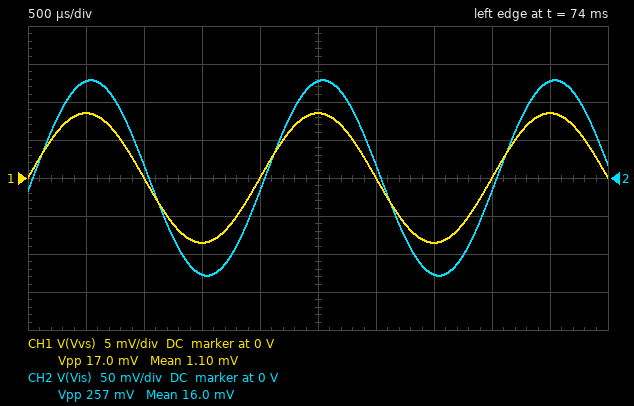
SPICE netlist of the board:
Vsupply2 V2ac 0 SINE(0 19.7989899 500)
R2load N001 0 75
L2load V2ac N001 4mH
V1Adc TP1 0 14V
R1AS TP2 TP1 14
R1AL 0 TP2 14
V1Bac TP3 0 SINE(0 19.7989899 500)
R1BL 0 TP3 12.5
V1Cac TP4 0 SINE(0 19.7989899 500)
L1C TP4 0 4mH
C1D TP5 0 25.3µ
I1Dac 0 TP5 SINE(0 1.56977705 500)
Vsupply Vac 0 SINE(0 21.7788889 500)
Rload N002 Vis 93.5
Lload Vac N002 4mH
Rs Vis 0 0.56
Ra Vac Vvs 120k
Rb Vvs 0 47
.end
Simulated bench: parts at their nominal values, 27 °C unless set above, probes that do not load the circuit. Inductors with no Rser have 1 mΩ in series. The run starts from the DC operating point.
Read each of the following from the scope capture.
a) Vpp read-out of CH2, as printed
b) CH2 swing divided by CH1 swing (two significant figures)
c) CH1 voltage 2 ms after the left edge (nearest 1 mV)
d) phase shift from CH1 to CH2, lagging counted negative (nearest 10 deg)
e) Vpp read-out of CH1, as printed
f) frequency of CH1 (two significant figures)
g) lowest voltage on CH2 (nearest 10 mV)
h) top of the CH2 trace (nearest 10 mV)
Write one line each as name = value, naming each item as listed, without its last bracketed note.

Vpp read-out of CH2, as printed = 257 mV
CH2 swing divided by CH1 swing = 15
CH1 voltage 2 ms after the left edge = 0 V
phase shift from CH1 to CH2, lagging counted negative = -10 deg
Vpp read-out of CH1, as printed = 17.0 mV
frequency of CH1 = 500 Hz
lowest voltage on CH2 = -130 mV
top of the CH2 trace = 130 mV
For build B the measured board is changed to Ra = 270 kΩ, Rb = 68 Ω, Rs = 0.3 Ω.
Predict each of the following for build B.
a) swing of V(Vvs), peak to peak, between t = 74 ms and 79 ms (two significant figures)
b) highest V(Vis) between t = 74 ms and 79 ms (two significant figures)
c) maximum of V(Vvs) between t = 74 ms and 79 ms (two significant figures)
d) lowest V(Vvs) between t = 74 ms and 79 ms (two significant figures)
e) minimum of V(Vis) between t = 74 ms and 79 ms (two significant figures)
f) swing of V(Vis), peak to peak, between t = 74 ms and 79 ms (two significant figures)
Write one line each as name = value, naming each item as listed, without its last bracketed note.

swing of V(Vvs), peak to peak, between t = 74 ms and 79 ms = 11 mV
highest V(Vis) between t = 74 ms and 79 ms = 69 mV
maximum of V(Vvs) between t = 74 ms and 79 ms = 5.5 mV
lowest V(Vvs) between t = 74 ms and 79 ms = -5.5 mV
minimum of V(Vis) between t = 74 ms and 79 ms = -69 mV
swing of V(Vis), peak to peak, between t = 74 ms and 79 ms = 140 mV
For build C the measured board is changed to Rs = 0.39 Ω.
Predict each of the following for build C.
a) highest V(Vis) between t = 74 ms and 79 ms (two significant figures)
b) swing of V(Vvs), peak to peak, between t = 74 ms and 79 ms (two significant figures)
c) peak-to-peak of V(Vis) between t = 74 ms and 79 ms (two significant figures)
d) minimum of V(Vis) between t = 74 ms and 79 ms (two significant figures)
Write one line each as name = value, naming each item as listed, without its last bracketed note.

highest V(Vis) between t = 74 ms and 79 ms = 90 mV
swing of V(Vvs), peak to peak, between t = 74 ms and 79 ms = 17 mV
peak-to-peak of V(Vis) between t = 74 ms and 79 ms = 180 mV
minimum of V(Vis) between t = 74 ms and 79 ms = -90 mV
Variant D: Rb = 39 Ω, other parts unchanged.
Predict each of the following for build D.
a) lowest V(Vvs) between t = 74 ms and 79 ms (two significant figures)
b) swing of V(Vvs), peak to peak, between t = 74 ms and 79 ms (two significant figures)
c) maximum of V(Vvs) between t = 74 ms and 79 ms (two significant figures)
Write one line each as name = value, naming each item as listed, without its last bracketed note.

lowest V(Vvs) between t = 74 ms and 79 ms = -7.1 mV
swing of V(Vvs), peak to peak, between t = 74 ms and 79 ms = 14 mV
maximum of V(Vvs) between t = 74 ms and 79 ms = 7.1 mV
